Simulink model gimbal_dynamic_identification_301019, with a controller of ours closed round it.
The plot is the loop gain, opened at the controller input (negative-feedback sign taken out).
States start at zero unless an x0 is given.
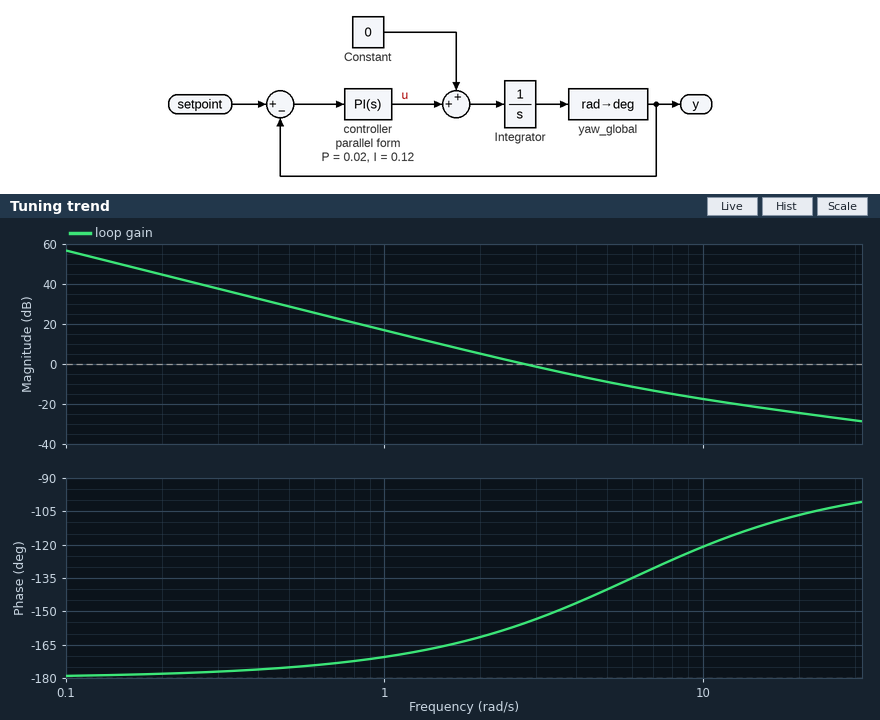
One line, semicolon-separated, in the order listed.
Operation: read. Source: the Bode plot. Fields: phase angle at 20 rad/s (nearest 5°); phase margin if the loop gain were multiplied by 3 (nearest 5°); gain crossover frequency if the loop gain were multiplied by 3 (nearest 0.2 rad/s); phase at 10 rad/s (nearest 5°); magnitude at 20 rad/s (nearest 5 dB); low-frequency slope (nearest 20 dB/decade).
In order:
-105°; 40°; 5.2 rad/s; -120°; -25 dB; -40 dB/decade
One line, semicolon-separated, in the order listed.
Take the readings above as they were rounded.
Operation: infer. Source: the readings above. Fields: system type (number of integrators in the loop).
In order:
2
